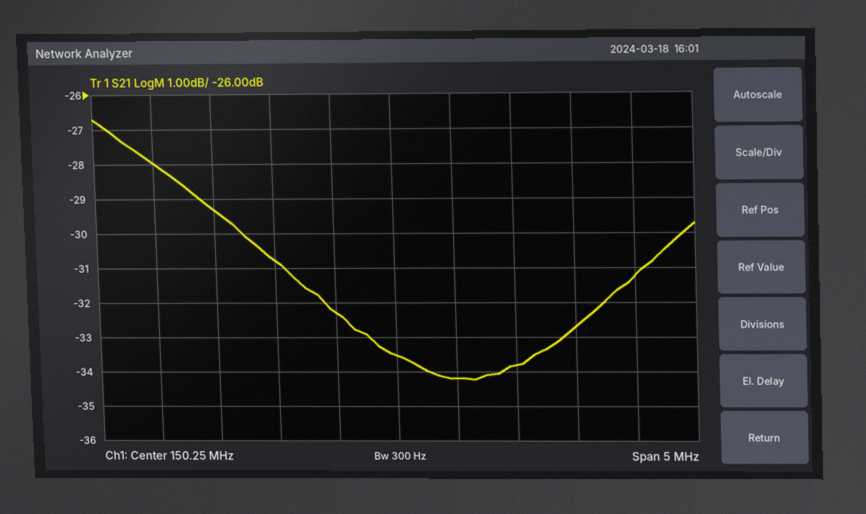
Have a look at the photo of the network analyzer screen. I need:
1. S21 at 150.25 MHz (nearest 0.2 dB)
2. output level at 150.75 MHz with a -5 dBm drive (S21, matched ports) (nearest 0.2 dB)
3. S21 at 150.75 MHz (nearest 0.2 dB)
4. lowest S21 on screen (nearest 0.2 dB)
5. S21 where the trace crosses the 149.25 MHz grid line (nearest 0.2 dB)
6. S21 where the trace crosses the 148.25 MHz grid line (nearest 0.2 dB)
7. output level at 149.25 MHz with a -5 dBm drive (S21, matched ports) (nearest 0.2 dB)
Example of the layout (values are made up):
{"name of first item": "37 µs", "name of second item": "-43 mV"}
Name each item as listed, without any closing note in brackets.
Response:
{"S21 at 150.25 MHz": "-33.6 dB", "output level at 150.75 MHz with a -5 dBm drive (S21, matched ports)": "-39.2 dBm", "S21 at 150.75 MHz": "-34.2 dB", "lowest S21 on screen": "-34.2 dB", "S21 where the trace crosses the 149.25 MHz grid line": "-30.8 dB", "S21 where the trace crosses the 148.25 MHz grid line": "-28.0 dB", "output level at 149.25 MHz with a -5 dBm drive (S21, matched ports)": "-35.8 dBm"}
